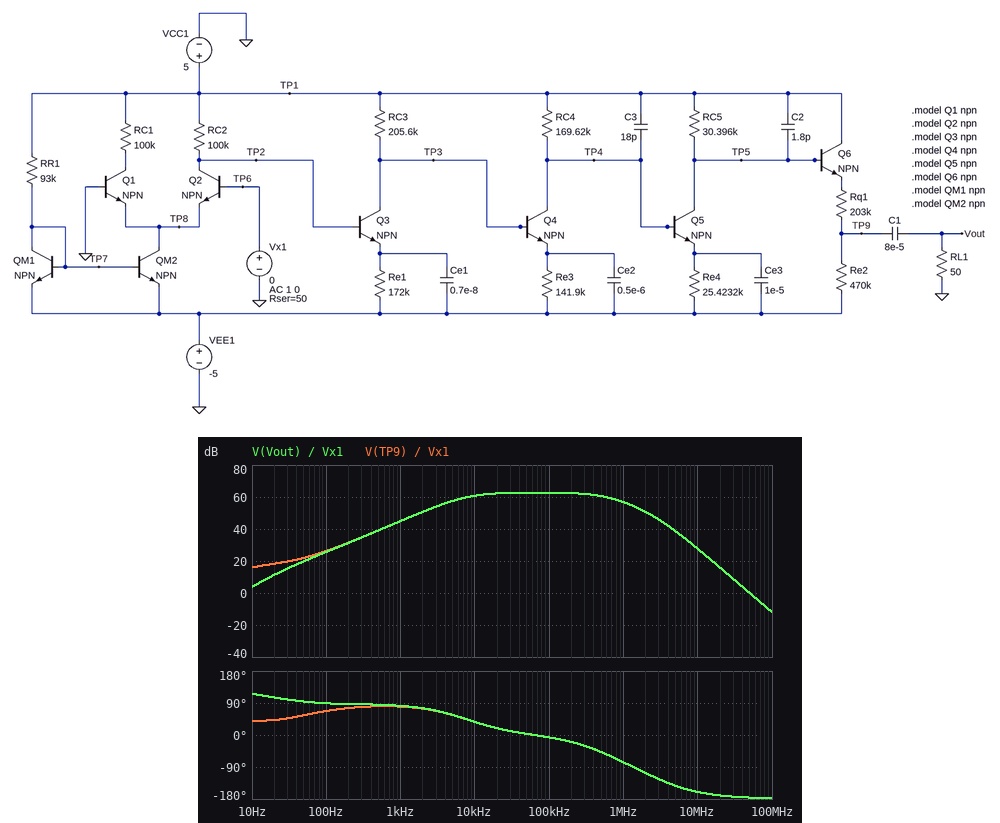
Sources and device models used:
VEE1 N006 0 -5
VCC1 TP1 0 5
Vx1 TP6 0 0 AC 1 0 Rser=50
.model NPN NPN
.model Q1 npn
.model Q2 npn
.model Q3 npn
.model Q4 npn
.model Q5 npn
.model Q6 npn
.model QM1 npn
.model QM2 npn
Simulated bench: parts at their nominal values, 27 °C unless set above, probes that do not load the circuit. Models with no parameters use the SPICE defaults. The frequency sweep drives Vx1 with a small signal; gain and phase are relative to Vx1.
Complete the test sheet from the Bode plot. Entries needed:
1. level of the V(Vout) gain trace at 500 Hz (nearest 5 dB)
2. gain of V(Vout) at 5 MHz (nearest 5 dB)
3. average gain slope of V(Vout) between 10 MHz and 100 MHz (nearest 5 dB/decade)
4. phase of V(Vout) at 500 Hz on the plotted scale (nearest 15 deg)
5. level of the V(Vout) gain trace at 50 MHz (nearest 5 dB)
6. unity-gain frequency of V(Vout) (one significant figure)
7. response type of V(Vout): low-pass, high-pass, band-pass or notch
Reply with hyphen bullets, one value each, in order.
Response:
- 40 dB
- 40 dB
- -40 dB/decade
- 90 deg
- 0 dB
- 50 MHz
- band-pass
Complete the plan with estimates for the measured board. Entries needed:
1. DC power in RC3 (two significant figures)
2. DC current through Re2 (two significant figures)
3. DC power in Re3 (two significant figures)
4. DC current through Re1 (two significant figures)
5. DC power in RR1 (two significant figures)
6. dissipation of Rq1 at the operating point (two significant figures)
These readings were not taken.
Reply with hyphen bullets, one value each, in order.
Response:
- 140 µW
- 6.4 µA
- 110 µW
- 26 µA
- 930 µW
- 8.3 µW
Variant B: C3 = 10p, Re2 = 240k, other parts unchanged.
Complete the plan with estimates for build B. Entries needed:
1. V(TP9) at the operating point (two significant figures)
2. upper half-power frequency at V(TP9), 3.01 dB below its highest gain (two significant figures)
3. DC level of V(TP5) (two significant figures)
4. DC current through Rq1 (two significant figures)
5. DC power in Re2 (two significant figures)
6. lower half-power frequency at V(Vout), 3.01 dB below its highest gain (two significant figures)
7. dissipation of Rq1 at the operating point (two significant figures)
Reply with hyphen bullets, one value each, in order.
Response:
- -2.7 V
- 1.0 MHz
- -49 mV
- 9.7 µA
- 23 µW
- 7.7 kHz
- 19 µW
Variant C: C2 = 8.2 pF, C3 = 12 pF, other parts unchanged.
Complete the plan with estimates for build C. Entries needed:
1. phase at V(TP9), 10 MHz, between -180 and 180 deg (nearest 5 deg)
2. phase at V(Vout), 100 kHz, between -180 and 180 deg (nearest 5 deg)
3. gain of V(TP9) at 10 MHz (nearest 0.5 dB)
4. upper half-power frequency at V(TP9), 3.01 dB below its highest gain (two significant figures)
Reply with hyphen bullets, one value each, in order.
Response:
- -170 deg
- -10 deg
- 18.5 dB
- 500 kHz
